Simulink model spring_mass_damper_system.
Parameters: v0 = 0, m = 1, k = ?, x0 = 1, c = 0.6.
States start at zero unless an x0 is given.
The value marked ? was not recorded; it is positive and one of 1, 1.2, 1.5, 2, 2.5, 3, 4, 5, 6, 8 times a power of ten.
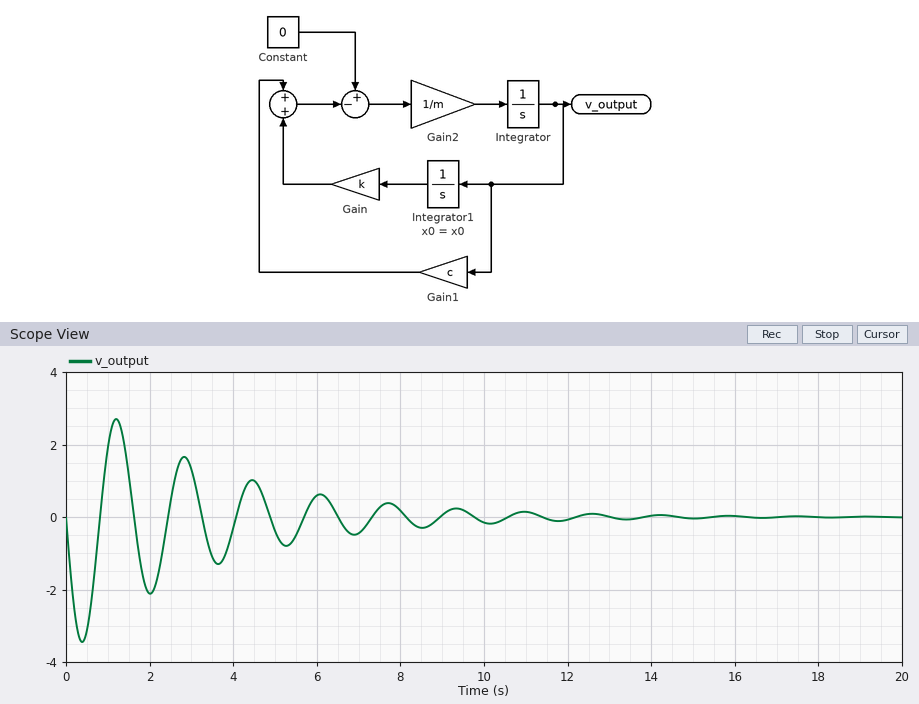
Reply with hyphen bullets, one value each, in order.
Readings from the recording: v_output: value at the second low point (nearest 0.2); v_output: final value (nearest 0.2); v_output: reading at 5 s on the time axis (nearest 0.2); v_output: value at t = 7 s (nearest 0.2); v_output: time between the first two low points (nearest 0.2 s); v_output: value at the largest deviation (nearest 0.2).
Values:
- -2.2
- 0.0
- -0.4
- -0.4
- 1.6 s
- -3.4
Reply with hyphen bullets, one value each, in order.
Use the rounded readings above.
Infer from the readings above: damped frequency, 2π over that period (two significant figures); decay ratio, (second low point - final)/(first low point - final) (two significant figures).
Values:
- 3.9 rad/s
- 0.65
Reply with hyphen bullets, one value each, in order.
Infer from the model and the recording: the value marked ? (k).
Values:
- 15
